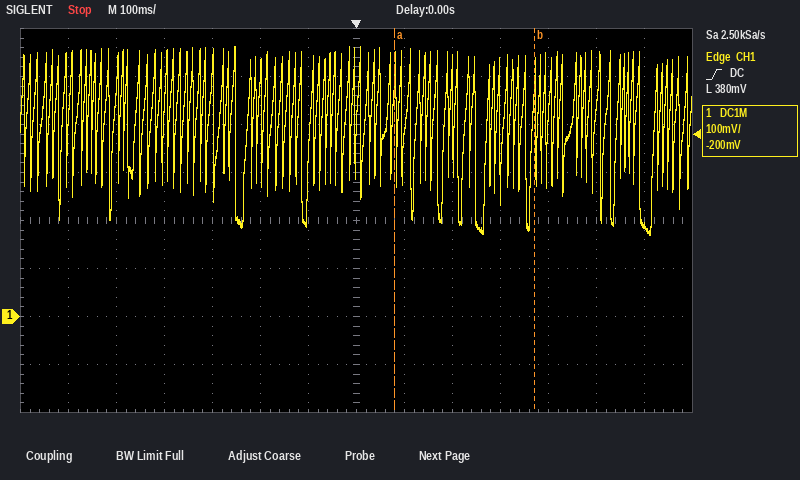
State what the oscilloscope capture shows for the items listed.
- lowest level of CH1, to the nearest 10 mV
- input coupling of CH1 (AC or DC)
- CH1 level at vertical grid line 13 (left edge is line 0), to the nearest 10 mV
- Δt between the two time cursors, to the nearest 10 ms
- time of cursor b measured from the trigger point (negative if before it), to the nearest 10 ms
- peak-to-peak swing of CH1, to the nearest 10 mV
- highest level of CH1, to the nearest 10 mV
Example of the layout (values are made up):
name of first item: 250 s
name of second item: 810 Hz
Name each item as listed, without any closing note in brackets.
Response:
lowest level of CH1, to the nearest 10 mV: 170 mV
input coupling of CH1: DC
CH1 level at vertical grid line 13 (left edge is line 0), to the nearest 10 mV: 190 mV
Δt between the two time cursors, to the nearest 10 ms: 290 ms
time of cursor b measured from the trigger point (negative if before it), to the nearest 10 ms: +370 ms
peak-to-peak swing of CH1, to the nearest 10 mV: 390 mV
highest level of CH1, to the nearest 10 mV: 560 mV
